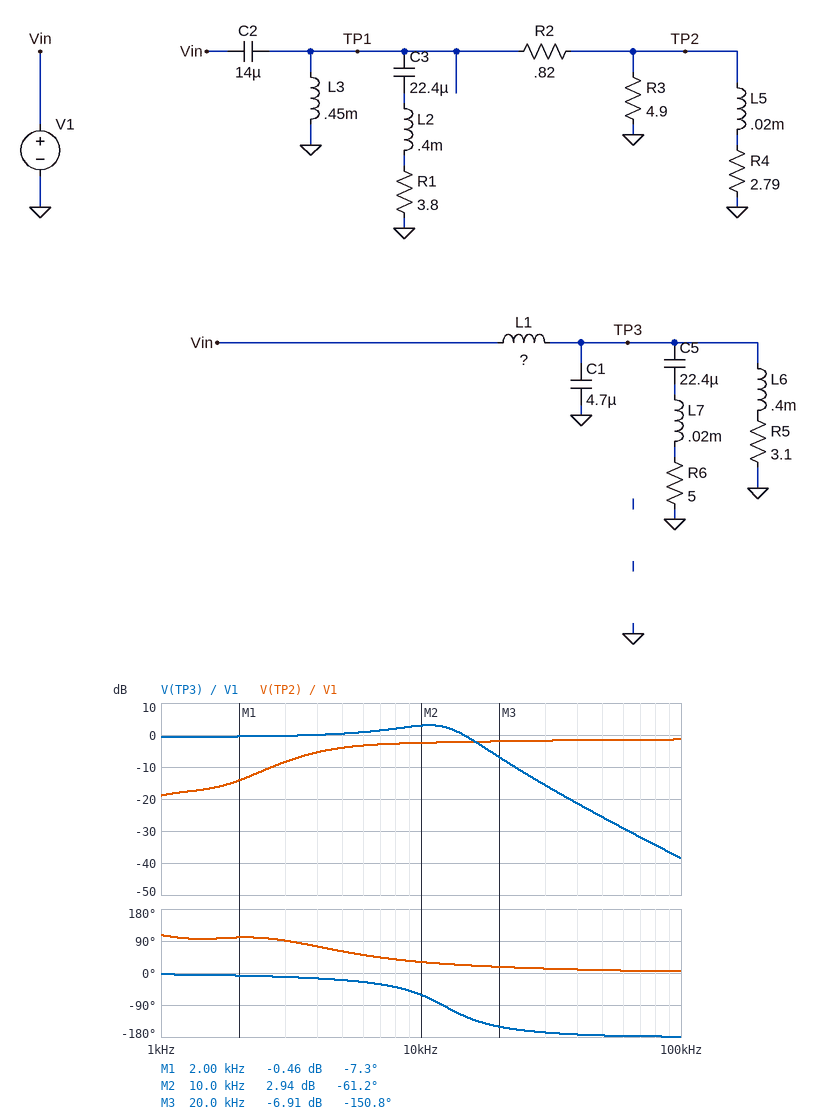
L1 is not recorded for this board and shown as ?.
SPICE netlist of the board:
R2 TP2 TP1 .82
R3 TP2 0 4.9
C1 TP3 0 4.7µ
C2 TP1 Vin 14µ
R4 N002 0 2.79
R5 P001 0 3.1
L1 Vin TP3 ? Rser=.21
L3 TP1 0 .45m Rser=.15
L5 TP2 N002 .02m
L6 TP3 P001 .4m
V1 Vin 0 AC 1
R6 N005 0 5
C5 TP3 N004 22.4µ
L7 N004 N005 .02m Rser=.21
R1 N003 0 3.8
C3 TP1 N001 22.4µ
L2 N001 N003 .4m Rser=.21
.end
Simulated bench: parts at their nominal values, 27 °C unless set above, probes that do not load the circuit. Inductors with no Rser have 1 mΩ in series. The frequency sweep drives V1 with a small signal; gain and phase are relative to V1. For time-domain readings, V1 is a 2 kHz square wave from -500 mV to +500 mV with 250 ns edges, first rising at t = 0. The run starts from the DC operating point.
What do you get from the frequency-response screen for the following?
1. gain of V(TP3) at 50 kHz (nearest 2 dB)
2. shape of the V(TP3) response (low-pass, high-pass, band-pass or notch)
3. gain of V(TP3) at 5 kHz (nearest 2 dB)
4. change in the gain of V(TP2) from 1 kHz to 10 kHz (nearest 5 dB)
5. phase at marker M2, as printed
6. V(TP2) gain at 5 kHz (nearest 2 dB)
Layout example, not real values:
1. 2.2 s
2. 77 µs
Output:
1. -26 dB
2. low-pass
3. 0 dB
4. 15 dB
5. -61.2 deg
6. -4 dB
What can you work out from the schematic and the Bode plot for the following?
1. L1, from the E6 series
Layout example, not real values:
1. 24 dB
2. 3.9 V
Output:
1. 47 µH
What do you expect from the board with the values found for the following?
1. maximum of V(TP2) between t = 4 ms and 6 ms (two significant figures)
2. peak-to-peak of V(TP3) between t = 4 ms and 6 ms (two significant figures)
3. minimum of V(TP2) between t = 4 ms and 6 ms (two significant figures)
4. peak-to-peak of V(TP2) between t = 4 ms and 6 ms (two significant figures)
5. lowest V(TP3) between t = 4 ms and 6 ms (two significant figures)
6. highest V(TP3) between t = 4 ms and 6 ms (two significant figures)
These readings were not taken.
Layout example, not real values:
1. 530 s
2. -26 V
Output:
1. 840 mV
2. 1.5 V
3. -840 mV
4. 1.7 V
5. -750 mV
6. 750 mV
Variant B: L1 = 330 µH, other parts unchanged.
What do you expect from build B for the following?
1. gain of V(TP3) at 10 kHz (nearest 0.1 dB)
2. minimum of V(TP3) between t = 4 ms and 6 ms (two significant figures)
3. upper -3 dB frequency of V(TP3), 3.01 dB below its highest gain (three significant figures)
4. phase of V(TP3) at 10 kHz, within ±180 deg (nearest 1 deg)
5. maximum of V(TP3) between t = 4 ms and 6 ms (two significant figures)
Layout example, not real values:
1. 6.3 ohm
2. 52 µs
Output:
1. -15.0 dB
2. -410 mV
3. 2.72 kHz
4. -133 deg
5. 410 mV
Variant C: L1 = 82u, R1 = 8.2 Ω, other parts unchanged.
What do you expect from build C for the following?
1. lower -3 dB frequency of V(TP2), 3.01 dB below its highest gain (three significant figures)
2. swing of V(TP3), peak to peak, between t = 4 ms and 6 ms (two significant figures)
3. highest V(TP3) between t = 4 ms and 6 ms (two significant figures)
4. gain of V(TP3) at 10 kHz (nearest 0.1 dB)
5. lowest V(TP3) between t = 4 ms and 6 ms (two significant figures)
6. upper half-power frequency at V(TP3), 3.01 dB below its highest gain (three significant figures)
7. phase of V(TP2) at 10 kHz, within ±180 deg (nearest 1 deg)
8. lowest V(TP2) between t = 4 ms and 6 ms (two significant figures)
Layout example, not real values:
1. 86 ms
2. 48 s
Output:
1. 5.04 kHz
2. 1.3 V
3. 630 mV
4. -0.6 dB
5. -630 mV
6. 11.2 kHz
7. 31 deg
8. -870 mV
